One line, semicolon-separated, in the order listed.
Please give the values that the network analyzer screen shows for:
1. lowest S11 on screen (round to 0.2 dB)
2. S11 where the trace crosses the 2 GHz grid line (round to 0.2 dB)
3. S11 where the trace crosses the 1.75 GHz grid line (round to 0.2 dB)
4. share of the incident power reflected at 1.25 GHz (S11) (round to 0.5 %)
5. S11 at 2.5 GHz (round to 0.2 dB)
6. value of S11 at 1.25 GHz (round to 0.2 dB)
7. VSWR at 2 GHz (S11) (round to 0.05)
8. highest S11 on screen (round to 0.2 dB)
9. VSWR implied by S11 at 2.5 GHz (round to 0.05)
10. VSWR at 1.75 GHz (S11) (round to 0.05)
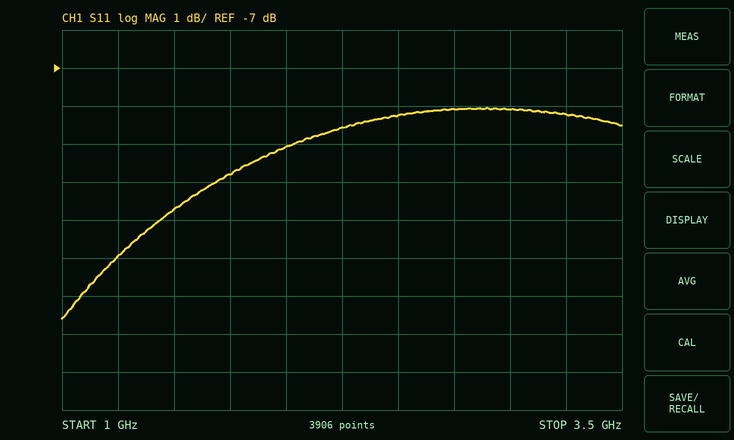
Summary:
-13.6 dB; -9.0 dB; -9.8 dB; 6.5 %; -8.2 dB; -12.0 dB; 2.10; -8.0 dB; 2.25; 1.95
